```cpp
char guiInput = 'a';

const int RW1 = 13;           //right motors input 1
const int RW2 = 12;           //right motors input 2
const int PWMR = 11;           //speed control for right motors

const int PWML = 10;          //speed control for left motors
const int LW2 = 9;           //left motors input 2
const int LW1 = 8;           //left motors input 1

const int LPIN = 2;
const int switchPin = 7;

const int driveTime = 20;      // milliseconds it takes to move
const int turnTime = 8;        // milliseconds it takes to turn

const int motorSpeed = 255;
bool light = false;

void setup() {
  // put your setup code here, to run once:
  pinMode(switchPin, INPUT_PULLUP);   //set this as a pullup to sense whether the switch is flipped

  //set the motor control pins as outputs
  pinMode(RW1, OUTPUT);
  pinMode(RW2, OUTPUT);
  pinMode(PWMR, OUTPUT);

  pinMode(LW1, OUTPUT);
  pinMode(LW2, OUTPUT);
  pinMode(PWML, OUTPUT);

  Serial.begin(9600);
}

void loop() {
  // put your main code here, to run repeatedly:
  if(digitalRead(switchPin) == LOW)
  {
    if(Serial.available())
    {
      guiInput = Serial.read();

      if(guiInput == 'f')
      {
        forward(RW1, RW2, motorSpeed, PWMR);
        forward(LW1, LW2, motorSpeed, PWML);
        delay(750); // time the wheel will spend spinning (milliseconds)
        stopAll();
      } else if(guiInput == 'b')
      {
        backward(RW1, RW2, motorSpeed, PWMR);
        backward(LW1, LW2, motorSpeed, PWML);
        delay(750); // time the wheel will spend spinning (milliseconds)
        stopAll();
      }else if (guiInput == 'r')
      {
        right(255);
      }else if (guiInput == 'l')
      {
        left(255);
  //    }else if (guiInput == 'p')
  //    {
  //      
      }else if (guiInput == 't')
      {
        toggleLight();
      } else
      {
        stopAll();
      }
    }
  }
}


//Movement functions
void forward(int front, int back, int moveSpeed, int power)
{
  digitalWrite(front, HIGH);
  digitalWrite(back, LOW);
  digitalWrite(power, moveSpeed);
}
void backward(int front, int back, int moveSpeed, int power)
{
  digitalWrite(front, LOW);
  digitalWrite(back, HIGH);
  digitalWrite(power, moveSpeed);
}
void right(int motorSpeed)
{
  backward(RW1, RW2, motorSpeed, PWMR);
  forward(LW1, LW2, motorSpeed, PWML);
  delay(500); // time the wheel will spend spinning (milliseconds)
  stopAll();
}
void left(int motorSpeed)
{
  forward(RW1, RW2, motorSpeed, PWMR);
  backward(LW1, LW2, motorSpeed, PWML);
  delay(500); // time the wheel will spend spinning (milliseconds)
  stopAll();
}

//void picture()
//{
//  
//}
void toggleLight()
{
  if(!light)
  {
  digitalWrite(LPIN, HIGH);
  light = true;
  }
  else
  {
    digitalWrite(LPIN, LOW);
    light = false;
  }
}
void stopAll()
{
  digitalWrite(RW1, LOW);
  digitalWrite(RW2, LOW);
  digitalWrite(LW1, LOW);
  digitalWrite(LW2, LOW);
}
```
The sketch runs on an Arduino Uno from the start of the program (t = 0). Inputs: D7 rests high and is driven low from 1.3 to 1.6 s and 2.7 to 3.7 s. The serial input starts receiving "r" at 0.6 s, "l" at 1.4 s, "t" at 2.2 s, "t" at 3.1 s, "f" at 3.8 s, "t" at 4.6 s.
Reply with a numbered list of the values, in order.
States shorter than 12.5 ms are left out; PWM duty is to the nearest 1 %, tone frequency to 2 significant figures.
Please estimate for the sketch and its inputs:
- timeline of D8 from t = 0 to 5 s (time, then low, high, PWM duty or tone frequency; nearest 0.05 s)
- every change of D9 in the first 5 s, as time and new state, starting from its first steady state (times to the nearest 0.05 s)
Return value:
1. 0 s low; 1.3 s high; 1.8 s low
2. 0 s low; 2.7 s high; 3.2 s low
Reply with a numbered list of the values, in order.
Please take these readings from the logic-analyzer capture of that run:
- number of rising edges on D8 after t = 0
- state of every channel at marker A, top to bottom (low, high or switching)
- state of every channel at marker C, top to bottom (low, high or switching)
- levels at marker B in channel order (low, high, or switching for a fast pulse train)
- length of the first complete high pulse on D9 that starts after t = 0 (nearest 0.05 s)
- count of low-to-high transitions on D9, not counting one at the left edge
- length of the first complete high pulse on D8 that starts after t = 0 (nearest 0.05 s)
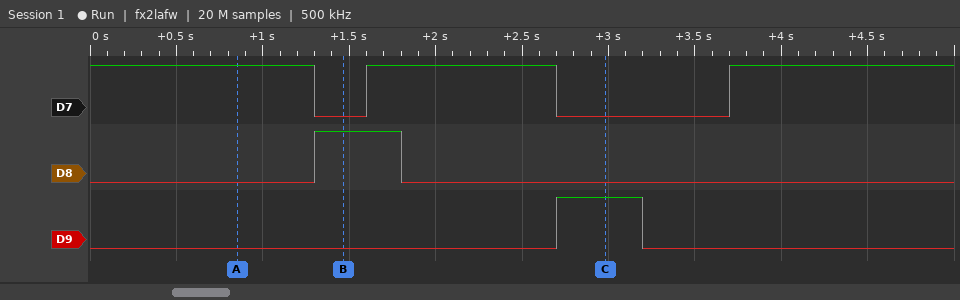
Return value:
1. 1
2. D7 high, D8 low, D9 low
3. D7 low, D8 low, D9 high
4. D7 low, D8 high, D9 low
5. 0.50 s
6. 1
7. 0.50 s
